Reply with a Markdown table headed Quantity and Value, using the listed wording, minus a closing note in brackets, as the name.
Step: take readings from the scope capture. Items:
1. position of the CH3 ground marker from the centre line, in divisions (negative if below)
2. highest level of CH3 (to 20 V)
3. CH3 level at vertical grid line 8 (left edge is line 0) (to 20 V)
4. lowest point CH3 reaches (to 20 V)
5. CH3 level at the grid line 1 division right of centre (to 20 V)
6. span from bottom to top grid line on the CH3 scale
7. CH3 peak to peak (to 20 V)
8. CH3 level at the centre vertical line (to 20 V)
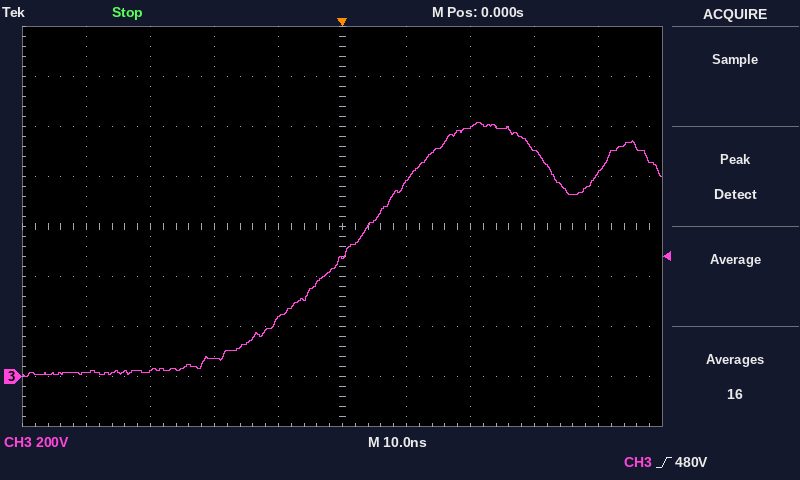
| Quantity | Value |
|---|---|
| position of the CH3 ground marker from the centre line, in divisions | -3.0 div |
| highest level of CH3 | 1.02 kV |
| CH3 level at vertical grid line 8 (left edge is line 0) | 900 V |
| lowest point CH3 reaches | 0 V |
| CH3 level at the grid line 1 division right of centre | 780 V |
| span from bottom to top grid line on the CH3 scale | 1.6 kV |
| CH3 peak to peak | 1.02 kV |
| CH3 level at the centre vertical line | 480 V |
